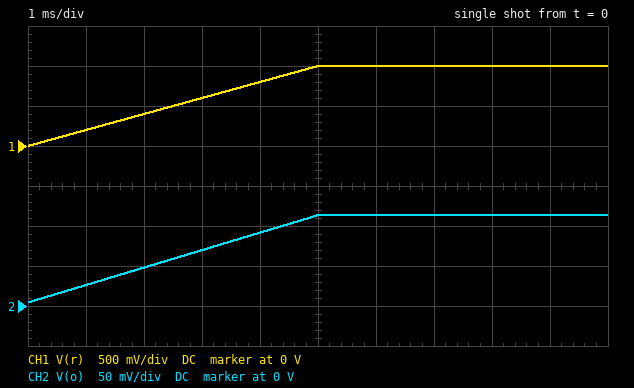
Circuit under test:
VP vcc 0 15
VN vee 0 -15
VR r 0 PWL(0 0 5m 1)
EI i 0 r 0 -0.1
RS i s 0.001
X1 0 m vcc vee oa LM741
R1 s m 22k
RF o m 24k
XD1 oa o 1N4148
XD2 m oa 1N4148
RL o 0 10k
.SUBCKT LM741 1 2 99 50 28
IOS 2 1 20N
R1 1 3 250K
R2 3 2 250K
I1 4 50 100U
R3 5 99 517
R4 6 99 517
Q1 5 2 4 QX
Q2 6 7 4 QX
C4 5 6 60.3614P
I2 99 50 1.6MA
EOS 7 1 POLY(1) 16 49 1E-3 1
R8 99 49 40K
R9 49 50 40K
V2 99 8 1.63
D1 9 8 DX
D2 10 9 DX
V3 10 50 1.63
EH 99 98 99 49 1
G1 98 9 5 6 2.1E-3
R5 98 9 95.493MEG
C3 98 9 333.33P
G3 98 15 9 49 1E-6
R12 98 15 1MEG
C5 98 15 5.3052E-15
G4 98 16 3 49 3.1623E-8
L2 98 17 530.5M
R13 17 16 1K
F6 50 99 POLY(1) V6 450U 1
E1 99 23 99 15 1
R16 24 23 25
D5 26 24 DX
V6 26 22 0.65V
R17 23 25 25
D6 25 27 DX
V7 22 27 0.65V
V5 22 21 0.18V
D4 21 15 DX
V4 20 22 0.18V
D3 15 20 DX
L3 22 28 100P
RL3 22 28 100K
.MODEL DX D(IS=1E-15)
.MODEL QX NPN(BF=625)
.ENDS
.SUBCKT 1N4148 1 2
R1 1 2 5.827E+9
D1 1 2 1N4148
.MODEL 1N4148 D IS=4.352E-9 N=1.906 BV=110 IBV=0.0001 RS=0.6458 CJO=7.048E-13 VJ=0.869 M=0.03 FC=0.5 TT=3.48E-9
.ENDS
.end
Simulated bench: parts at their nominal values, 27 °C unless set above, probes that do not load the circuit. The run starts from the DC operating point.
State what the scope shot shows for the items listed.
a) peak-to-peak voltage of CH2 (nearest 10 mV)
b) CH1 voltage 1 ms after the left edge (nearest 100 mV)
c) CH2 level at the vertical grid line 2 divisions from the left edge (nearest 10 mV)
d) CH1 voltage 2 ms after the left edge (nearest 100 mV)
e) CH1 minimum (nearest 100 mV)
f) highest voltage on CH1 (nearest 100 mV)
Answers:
110 mV
200 mV
50 mV
400 mV
0 V
1.0 V
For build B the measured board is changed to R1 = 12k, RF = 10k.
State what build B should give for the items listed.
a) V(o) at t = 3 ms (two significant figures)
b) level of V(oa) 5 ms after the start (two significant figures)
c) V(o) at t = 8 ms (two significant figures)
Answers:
53 mV
490 mV
86 mV
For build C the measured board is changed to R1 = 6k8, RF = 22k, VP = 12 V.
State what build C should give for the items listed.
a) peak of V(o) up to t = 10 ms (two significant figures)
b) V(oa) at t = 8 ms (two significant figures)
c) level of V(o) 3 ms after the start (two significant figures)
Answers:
330 mV
790 mV
200 mV
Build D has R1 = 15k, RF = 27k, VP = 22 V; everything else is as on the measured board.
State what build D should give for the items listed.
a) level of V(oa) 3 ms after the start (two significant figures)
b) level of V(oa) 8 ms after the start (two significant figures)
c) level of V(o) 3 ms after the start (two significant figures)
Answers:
520 mV
610 mV
110 mV
